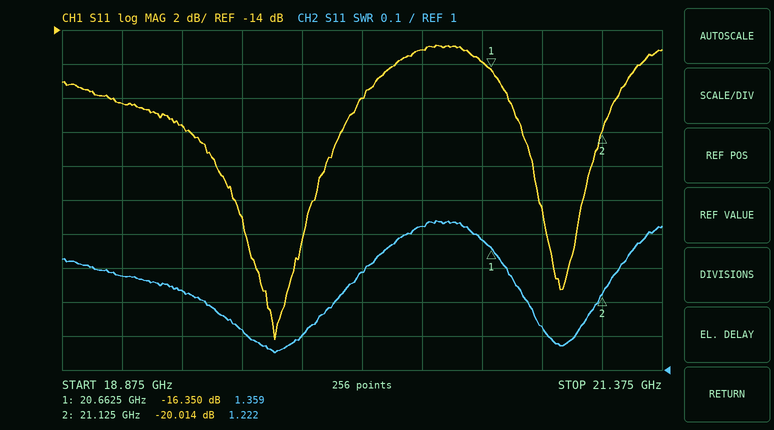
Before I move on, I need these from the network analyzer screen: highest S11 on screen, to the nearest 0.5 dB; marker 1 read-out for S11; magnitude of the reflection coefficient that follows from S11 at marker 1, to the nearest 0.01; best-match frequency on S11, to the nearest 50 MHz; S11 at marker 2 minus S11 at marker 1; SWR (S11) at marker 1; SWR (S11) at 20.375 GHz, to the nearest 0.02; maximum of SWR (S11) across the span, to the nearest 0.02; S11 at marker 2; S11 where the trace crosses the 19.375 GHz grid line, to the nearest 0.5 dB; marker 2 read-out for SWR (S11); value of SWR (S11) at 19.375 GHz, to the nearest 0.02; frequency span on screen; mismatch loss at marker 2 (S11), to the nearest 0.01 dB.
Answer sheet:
-15.0 dB
-16.350 dB
0.15
19.75 GHz
-3.664 dB
1.359
1.42
1.44
-20.014 dB
-19.5 dB
1.222
1.24
2.5 GHz
0.04 dB
